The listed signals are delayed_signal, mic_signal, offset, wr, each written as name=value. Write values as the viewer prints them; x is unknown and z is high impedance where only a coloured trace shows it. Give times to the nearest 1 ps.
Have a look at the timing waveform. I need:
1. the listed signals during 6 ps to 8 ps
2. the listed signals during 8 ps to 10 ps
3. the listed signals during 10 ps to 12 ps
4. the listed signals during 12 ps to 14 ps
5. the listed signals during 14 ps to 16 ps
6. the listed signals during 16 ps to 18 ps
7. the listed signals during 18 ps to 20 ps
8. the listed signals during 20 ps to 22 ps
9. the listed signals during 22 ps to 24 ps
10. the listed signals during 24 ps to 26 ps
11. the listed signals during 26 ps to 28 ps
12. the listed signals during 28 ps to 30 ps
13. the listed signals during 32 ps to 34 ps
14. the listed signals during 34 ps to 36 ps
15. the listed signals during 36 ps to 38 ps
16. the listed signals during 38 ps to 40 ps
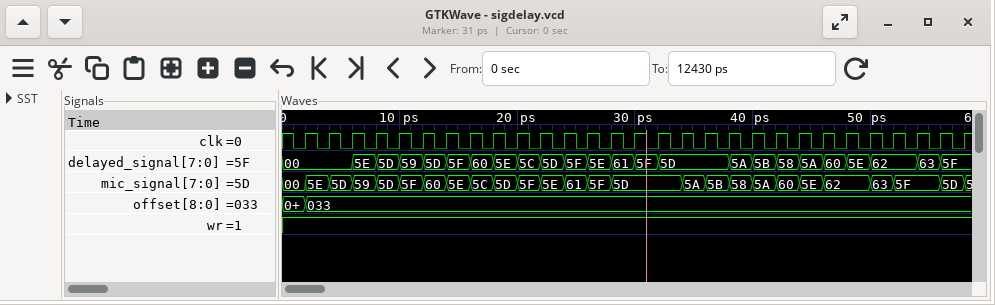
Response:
delayed_signal=5E, mic_signal=59, offset=033, wr=1
delayed_signal=5D, mic_signal=5D, offset=033, wr=1
delayed_signal=59, mic_signal=5F, offset=033, wr=1
delayed_signal=5D, mic_signal=60, offset=033, wr=1
delayed_signal=5F, mic_signal=5E, offset=033, wr=1
delayed_signal=60, mic_signal=5C, offset=033, wr=1
delayed_signal=5E, mic_signal=5D, offset=033, wr=1
delayed_signal=5C, mic_signal=5F, offset=033, wr=1
delayed_signal=5D, mic_signal=5E, offset=033, wr=1
delayed_signal=5F, mic_signal=61, offset=033, wr=1
delayed_signal=5E, mic_signal=5F, offset=033, wr=1
delayed_signal=61, mic_signal=5D, offset=033, wr=1
delayed_signal=5D, mic_signal=5D, offset=033, wr=1
delayed_signal=5D, mic_signal=5A, offset=033, wr=1
delayed_signal=5D, mic_signal=5B, offset=033, wr=1
delayed_signal=5A, mic_signal=58, offset=033, wr=1
